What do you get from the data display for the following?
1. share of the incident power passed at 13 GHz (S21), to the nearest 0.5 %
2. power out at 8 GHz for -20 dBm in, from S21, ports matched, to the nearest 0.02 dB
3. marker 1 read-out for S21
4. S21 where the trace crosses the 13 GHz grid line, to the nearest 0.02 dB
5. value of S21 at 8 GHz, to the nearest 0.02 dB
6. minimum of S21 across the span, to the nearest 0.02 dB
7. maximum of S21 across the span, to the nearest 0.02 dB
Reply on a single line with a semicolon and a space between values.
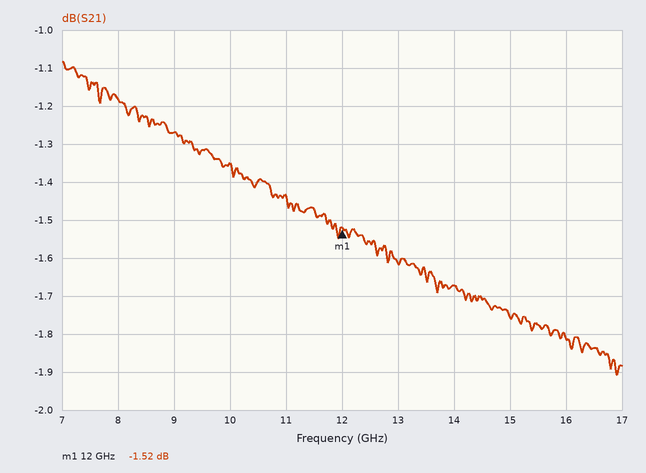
69.0 %; -21.18 dBm; -1.52 dB; -1.62 dB; -1.18 dB; -1.90 dB; -1.08 dB
